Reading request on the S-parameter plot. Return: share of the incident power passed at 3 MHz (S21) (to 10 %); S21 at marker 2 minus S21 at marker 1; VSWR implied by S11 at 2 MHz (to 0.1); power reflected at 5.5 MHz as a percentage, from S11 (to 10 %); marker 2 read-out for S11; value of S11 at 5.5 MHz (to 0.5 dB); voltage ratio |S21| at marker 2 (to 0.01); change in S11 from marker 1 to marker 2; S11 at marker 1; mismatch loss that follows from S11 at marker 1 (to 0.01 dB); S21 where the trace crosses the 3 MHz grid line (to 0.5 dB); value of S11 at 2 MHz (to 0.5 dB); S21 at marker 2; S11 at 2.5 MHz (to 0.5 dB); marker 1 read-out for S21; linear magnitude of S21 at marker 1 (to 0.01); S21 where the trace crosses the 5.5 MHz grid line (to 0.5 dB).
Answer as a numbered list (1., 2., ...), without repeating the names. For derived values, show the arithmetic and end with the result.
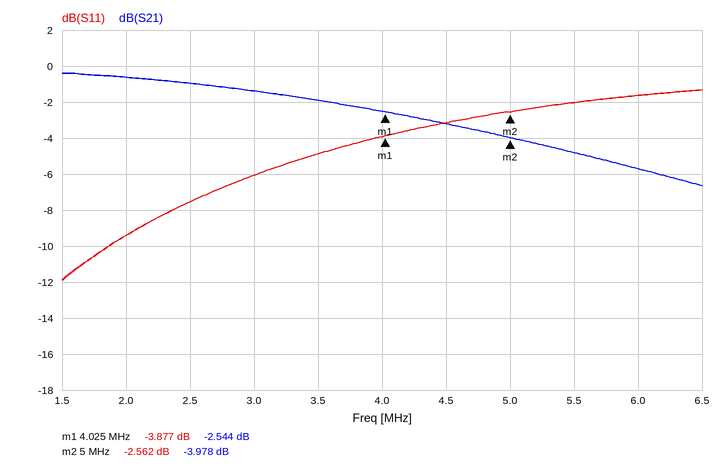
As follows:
1. 10^(-1.5/10) ≈ 70.8 %, so 70 % to the nearest 10 %
2. -3.978 − (-2.544) = -1.434 dB
3. |Γ| = 10^(-9.5/20) = 0.3350; VSWR = (1 + 0.3350)/(1 − 0.3350) ≈ 2.0
4. 10^(-2/10) ≈ 63.1 %, so 60 % to the nearest 10 %
5. -2.562 dB
6. -2.0 dB
7. 10^(-3.978/20) ≈ 0.63
8. -2.562 − (-3.877) = 1.315 dB
9. -3.877 dB
10. −10 log10(1 − 10^(-3.877/10)) ≈ 2.29 dB
11. -1.5 dB
12. -9.5 dB
13. -3.978 dB
14. -7.5 dB
15. -2.544 dB
16. 10^(-2.544/20) ≈ 0.75
17. -5.0 dB
